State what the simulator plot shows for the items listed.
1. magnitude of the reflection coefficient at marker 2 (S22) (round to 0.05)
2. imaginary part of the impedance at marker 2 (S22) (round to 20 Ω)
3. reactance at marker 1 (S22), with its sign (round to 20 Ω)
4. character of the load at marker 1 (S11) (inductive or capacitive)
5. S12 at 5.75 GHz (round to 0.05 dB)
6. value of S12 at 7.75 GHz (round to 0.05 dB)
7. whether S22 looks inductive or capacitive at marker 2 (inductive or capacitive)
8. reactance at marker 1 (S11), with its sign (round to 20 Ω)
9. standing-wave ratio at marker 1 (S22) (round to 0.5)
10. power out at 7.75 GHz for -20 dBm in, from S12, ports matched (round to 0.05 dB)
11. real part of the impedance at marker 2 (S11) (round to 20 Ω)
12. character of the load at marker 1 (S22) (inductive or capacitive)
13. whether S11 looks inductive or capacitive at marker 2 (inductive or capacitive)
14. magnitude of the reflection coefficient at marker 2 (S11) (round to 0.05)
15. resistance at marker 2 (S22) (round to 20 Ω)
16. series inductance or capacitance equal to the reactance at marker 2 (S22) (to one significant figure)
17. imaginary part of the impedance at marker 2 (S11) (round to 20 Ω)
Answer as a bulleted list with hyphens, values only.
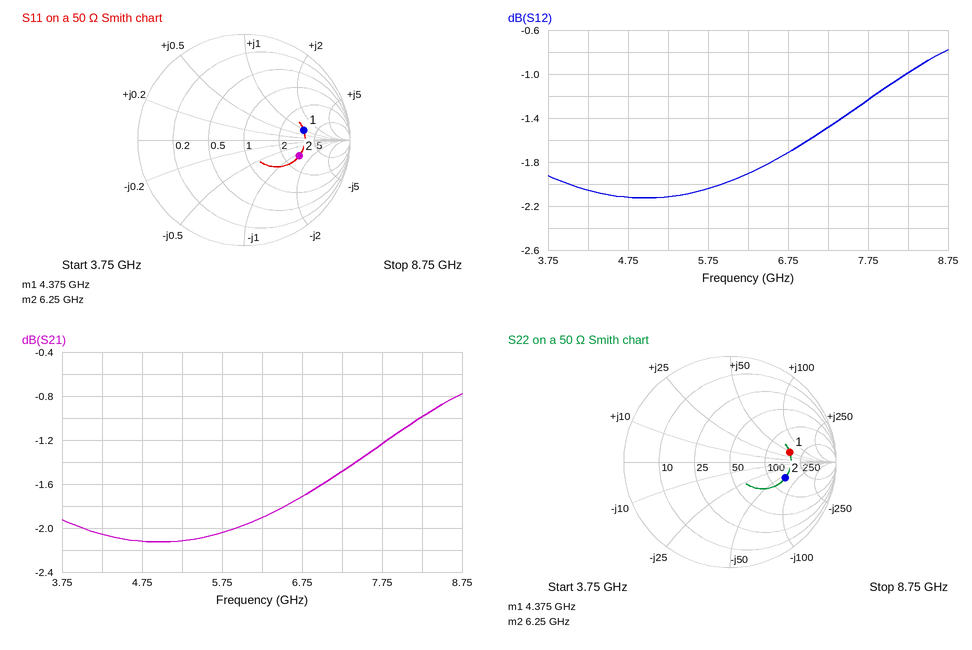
- 0.55
- -60 Ω
- +40 Ω
- inductive
- -2.05 dB
- -1.25 dB
- capacitive
- +40 Ω
- 3.5
- -21.25 dBm
- 140 Ω
- inductive
- capacitive
- 0.55
- 140 Ω
- 400 fF
- -60 Ω
